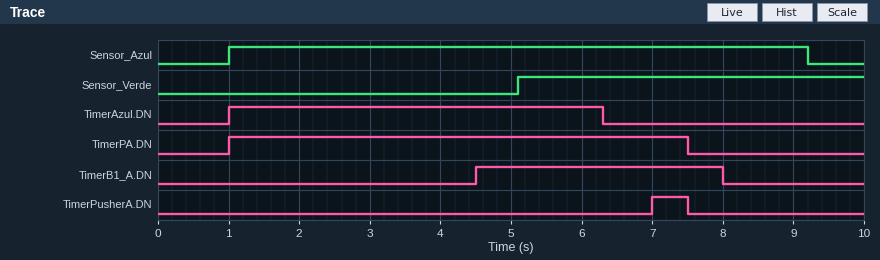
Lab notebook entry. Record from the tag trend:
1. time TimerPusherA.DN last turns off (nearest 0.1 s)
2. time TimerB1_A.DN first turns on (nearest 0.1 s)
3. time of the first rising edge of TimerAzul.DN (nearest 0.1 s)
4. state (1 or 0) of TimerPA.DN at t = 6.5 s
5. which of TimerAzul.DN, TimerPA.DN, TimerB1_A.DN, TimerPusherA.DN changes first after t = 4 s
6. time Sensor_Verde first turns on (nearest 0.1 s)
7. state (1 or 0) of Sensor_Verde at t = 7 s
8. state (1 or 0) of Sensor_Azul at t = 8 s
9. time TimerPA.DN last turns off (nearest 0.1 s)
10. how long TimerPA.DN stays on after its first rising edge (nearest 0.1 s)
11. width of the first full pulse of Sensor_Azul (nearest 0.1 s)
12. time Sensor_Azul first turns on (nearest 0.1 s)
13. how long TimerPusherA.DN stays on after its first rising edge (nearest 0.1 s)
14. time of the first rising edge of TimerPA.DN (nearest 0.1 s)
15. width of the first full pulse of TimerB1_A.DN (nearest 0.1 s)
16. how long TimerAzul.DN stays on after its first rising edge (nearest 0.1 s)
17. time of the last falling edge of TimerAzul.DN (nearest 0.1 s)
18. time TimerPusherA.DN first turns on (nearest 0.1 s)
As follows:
7.5 s
4.5 s
1.0 s
1
TimerB1_A.DN
5.1 s
1
1
7.5 s
6.5 s
8.2 s
1.0 s
0.5 s
1.0 s
3.5 s
5.3 s
6.3 s
7.0 s
